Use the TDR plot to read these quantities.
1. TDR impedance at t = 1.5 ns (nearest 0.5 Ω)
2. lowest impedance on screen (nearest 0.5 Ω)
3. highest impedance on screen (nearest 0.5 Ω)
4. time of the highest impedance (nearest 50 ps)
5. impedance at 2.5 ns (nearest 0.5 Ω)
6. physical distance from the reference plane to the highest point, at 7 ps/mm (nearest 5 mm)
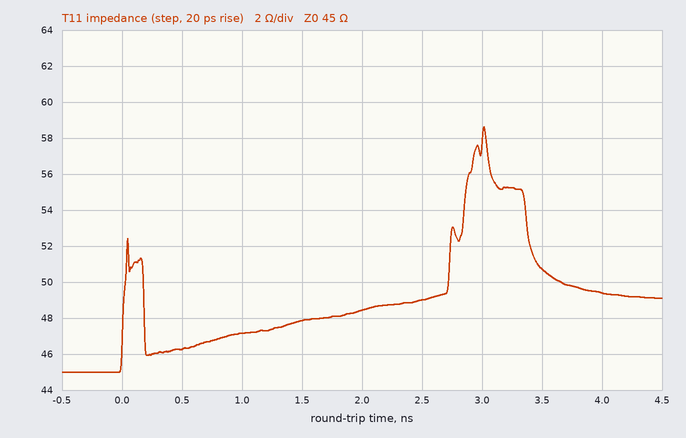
48.0 Ω
45.0 Ω
58.5 Ω
3.00 ns
49.0 Ω
215 mm
